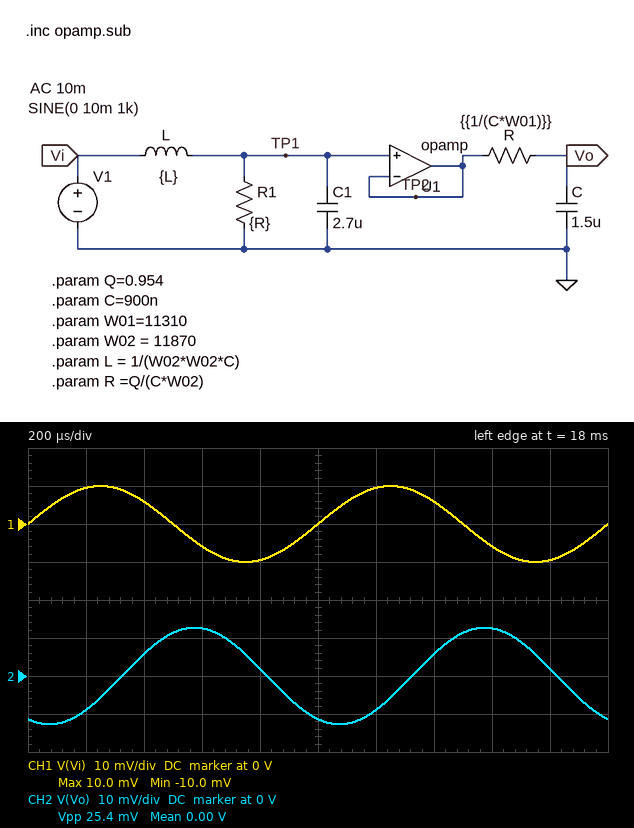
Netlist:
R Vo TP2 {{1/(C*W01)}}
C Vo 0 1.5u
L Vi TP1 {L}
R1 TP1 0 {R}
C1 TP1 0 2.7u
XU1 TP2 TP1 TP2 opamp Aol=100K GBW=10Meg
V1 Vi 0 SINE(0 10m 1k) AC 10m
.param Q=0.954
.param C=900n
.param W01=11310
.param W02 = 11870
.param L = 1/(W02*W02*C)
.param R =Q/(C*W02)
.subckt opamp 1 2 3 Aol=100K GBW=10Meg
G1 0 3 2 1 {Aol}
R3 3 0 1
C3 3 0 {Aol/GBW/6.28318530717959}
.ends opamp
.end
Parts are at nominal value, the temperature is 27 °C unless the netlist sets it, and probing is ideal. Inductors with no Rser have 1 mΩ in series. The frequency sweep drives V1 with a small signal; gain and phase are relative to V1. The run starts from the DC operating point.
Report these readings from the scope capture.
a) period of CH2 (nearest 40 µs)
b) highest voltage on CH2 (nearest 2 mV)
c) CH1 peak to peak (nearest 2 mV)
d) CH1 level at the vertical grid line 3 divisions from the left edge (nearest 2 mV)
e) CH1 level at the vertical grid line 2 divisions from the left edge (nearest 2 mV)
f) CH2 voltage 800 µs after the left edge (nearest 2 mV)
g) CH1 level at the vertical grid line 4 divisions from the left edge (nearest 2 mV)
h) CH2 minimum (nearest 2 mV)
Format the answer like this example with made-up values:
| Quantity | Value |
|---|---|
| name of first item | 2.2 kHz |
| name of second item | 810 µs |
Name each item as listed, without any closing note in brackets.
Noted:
| Quantity | Value |
|---|---|
| period of CH2 | 1.00 ms |
| highest voltage on CH2 | 12 mV |
| CH1 peak to peak | 20 mV |
| CH1 level at the vertical grid line 3 divisions from the left edge | -6 mV |
| CH1 level at the vertical grid line 2 divisions from the left edge | 6 mV |
| CH2 voltage 800 µs after the left edge | 2 mV |
| CH1 level at the vertical grid line 4 divisions from the left edge | -10 mV |
| CH2 minimum | -12 mV |
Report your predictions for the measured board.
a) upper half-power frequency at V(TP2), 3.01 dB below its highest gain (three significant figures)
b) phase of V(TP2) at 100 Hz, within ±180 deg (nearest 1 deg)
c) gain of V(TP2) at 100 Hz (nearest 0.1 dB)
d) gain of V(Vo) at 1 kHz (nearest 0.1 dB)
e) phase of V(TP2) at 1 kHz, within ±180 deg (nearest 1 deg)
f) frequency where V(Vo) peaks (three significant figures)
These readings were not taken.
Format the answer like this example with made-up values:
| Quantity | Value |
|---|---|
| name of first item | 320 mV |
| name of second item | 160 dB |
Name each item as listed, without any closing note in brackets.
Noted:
| Quantity | Value |
|---|---|
| upper half-power frequency at V(TP2), 3.01 dB below its highest gain | 1.29 kHz |
| phase of V(TP2) at 100 Hz, within ±180 deg | -3 deg |
| gain of V(TP2) at 100 Hz | 0.1 dB |
| gain of V(Vo) at 1 kHz | 2.1 dB |
| phase of V(TP2) at 1 kHz, within ±180 deg | -74 deg |
| frequency where V(Vo) peaks | 923 Hz |
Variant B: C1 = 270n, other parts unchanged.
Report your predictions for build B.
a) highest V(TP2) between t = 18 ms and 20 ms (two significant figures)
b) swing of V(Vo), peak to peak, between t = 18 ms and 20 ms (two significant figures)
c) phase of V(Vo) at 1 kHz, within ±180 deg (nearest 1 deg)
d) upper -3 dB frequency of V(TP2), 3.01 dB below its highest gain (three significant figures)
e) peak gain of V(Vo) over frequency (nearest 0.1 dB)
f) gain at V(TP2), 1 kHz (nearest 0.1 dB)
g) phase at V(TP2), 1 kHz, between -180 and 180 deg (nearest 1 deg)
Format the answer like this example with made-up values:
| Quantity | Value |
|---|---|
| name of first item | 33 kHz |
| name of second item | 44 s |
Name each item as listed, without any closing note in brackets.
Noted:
| Quantity | Value |
|---|---|
| highest V(TP2) between t = 18 ms and 20 ms | 9.3 mV |
| swing of V(Vo), peak to peak, between t = 18 ms and 20 ms | 14 mV |
| phase of V(Vo) at 1 kHz, within ±180 deg | -74 deg |
| upper -3 dB frequency of V(TP2), 3.01 dB below its highest gain | 2.36 kHz |
| peak gain of V(Vo) over frequency | 0 dB |
| gain at V(TP2), 1 kHz | -0.6 dB |
| phase at V(TP2), 1 kHz, between -180 and 180 deg | -31 deg |
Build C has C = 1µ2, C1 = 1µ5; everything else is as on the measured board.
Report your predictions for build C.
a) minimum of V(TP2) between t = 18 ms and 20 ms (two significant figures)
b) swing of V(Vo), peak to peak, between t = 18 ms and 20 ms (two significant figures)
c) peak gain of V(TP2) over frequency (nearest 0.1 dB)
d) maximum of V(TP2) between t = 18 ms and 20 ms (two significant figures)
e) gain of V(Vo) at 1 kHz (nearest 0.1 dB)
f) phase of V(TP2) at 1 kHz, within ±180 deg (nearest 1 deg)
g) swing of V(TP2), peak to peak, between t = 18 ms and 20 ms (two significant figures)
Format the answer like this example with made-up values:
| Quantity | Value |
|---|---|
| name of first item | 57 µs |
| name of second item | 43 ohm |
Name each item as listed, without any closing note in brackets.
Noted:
| Quantity | Value |
|---|---|
| minimum of V(TP2) between t = 18 ms and 20 ms | -13 mV |
| swing of V(Vo), peak to peak, between t = 18 ms and 20 ms | 21 mV |
| peak gain of V(TP2) over frequency | 2.6 dB |
| maximum of V(TP2) between t = 18 ms and 20 ms | 13 mV |
| gain of V(Vo) at 1 kHz | 0.4 dB |
| phase of V(TP2) at 1 kHz, within ±180 deg | -46 deg |
| swing of V(TP2), peak to peak, between t = 18 ms and 20 ms | 26 mV |
